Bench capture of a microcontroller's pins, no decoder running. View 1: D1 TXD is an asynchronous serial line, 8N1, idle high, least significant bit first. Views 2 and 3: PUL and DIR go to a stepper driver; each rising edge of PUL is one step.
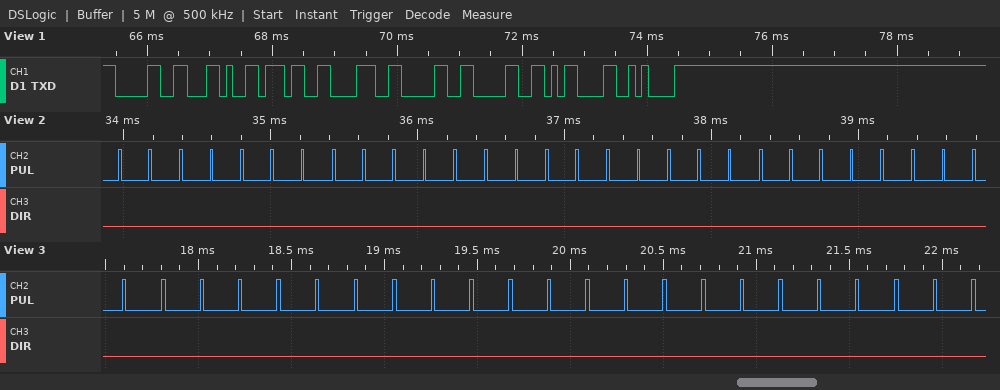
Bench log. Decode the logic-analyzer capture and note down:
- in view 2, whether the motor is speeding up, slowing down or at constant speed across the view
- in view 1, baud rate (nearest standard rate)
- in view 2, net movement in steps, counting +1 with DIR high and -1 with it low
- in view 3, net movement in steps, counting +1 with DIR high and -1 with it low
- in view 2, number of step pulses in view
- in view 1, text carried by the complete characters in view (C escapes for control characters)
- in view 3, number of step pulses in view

constant speed
9600 baud
-29
-23
29
"0,7800\r\n"
23
